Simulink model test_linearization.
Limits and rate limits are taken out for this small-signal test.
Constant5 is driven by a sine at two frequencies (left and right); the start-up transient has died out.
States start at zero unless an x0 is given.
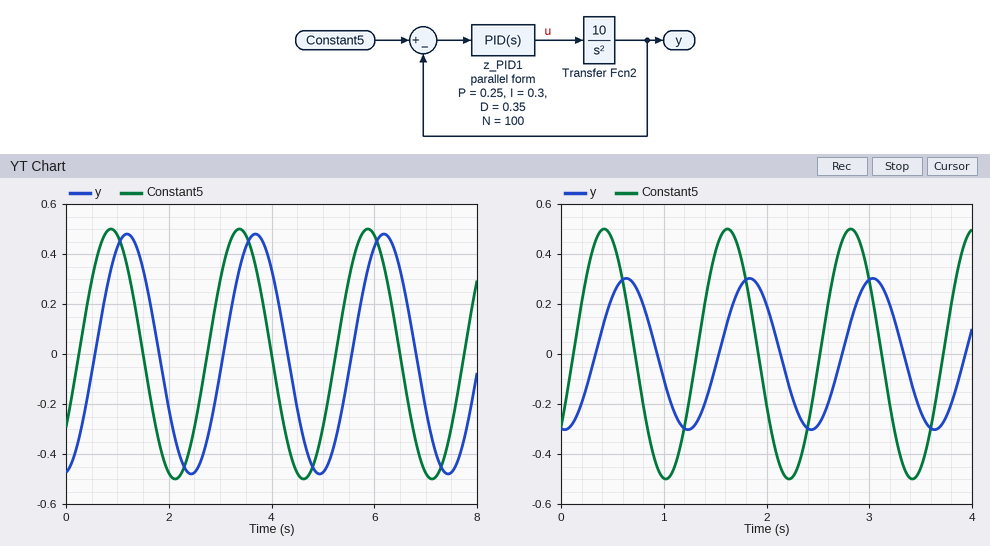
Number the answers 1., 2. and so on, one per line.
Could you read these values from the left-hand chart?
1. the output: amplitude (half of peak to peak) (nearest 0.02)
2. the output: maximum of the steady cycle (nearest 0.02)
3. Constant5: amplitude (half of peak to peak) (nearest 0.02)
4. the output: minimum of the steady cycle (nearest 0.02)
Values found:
1. 0.48
2. 0.48
3. 0.50
4. -0.48
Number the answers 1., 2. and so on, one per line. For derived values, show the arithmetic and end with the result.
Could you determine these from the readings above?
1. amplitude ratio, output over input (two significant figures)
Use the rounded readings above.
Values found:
1. 0.48 / 0.5 = 0.96
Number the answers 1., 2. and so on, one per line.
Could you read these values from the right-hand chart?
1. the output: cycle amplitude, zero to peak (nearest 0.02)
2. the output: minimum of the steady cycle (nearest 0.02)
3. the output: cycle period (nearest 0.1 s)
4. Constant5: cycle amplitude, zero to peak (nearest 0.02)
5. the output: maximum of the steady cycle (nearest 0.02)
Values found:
1. 0.30
2. -0.30
3. 1.2 s
4. 0.50
5. 0.30
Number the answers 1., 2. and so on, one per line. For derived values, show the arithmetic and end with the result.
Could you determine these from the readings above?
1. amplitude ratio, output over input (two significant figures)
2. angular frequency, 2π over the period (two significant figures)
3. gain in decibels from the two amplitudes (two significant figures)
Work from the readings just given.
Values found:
1. 0.3 / 0.5 = 0.60
2. 2π / 1.2 = 5.2 rad/s
3. 20 log10(0.3 / 0.5) = -4.4 dB
